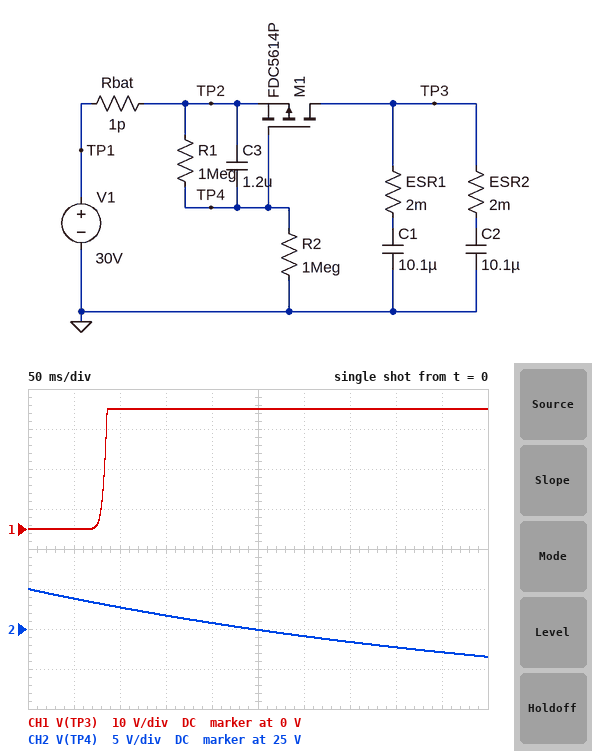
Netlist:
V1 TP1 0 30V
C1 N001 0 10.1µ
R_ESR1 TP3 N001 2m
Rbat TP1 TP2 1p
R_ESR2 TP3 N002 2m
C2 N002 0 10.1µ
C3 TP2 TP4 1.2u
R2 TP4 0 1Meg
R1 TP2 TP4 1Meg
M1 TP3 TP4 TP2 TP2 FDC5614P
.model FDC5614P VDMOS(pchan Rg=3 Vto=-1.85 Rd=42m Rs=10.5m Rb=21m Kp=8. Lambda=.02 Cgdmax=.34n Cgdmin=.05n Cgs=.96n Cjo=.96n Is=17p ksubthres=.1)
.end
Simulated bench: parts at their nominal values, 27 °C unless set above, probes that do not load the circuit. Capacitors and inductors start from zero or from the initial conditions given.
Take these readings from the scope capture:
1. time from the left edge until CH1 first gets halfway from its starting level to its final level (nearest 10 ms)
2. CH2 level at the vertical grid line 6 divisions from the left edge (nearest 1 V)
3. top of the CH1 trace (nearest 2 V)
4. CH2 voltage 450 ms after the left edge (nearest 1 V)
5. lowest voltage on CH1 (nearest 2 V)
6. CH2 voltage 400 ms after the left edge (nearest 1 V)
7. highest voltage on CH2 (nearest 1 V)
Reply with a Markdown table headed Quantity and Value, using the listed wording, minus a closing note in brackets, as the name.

| Quantity | Value |
|---|---|
| time from the left edge until CH1 first gets halfway from its starting level to its final level | 80 ms |
| CH2 level at the vertical grid line 6 divisions from the left edge | 24 V |
| top of the CH1 trace | 30 V |
| CH2 voltage 450 ms after the left edge | 22 V |
| lowest voltage on CH1 | 0 V |
| CH2 voltage 400 ms after the left edge | 23 V |
| highest voltage on CH2 | 30 V |
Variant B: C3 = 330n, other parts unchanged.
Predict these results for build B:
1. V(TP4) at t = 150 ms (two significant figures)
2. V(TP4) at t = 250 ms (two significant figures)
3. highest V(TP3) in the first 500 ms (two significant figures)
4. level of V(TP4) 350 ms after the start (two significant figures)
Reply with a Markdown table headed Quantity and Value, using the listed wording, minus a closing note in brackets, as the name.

| Quantity | Value |
|---|---|
| V(TP4) at t = 150 ms | 21 V |
| V(TP4) at t = 250 ms | 18 V |
| highest V(TP3) in the first 500 ms | 30 V |
| level of V(TP4) 350 ms after the start | 17 V |
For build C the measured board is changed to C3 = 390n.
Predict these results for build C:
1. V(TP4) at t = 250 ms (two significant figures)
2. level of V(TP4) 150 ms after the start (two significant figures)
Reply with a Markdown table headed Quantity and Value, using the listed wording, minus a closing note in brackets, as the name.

| Quantity | Value |
|---|---|
| V(TP4) at t = 250 ms | 19 V |
| level of V(TP4) 150 ms after the start | 22 V |
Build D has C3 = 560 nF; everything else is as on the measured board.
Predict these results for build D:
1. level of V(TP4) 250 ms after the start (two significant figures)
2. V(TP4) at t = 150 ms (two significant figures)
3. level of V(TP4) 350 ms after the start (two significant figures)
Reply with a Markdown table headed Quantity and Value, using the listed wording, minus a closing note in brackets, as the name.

| Quantity | Value |
|---|---|
| level of V(TP4) 250 ms after the start | 21 V |
| V(TP4) at t = 150 ms | 24 V |
| level of V(TP4) 350 ms after the start | 19 V |
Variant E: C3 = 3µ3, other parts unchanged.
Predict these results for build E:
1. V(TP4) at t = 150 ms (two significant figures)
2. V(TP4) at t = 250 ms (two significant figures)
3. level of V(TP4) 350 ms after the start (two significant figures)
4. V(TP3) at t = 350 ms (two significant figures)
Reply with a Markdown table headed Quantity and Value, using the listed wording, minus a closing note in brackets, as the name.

| Quantity | Value |
|---|---|
| V(TP4) at t = 150 ms | 29 V |
| V(TP4) at t = 250 ms | 28 V |
| level of V(TP4) 350 ms after the start | 27 V |
| V(TP3) at t = 350 ms | 30 V |
